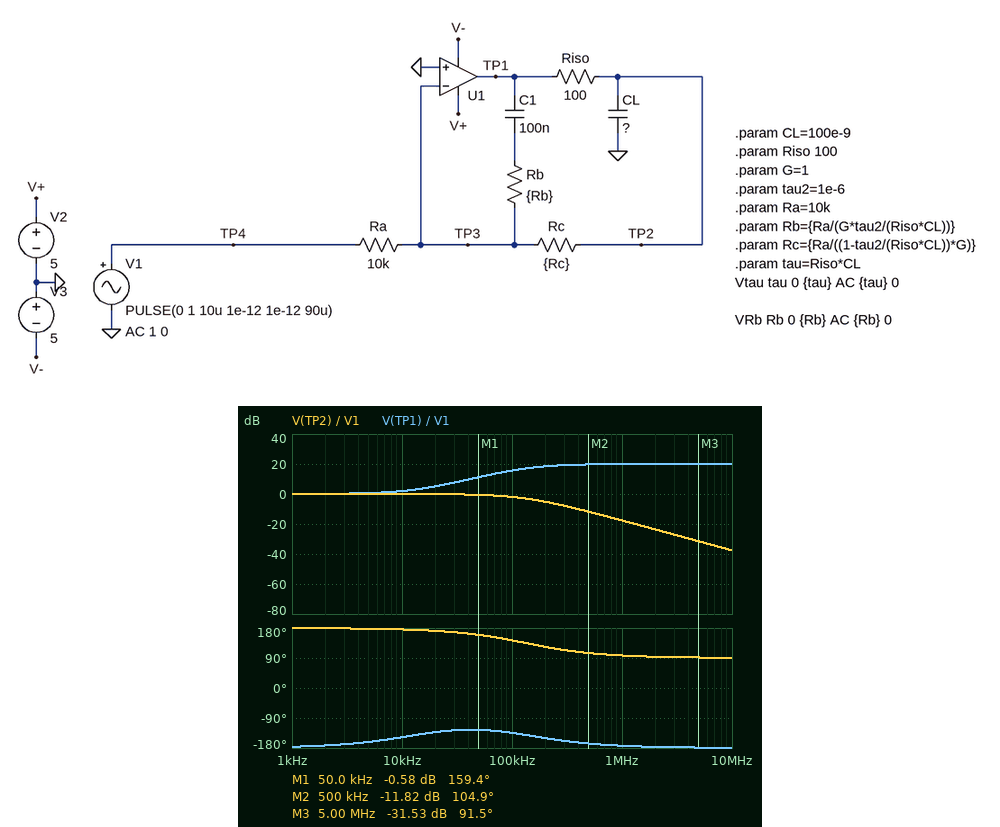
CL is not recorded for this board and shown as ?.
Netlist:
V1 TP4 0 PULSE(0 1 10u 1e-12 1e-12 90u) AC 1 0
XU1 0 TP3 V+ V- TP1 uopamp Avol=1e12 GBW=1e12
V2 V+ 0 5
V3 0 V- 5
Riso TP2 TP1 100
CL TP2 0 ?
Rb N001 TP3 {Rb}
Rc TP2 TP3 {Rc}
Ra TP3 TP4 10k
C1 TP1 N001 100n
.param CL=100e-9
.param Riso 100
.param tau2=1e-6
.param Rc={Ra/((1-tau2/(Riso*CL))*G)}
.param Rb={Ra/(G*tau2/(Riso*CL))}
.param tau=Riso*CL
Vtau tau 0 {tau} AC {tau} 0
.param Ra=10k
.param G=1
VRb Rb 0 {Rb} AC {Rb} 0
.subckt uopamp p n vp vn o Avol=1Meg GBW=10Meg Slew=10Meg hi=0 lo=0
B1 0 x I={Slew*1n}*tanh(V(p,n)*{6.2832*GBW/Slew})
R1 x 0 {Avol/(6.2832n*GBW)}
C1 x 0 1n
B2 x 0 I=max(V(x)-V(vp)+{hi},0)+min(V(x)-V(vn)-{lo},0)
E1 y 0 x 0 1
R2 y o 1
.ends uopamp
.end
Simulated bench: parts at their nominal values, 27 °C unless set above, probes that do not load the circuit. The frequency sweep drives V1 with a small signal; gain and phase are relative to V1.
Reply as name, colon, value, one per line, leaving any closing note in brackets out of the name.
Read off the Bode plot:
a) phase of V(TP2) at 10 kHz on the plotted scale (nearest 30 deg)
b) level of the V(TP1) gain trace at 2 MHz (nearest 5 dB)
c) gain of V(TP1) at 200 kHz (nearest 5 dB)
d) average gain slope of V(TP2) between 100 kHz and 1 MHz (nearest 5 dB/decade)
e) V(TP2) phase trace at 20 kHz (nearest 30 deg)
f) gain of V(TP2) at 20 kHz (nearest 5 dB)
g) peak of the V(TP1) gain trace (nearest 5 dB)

phase of V(TP2) at 10 kHz on the plotted scale: 180 deg
level of the V(TP1) gain trace at 2 MHz: 20 dB
gain of V(TP1) at 200 kHz: 20 dB
average gain slope of V(TP2) between 100 kHz and 1 MHz: -15 dB/decade
V(TP2) phase trace at 20 kHz: 180 deg
gain of V(TP2) at 20 kHz: 0 dB
peak of the V(TP1) gain trace: 20 dB
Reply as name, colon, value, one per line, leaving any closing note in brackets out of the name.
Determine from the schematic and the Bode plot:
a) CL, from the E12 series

CL, from the E12 series: 120 nF
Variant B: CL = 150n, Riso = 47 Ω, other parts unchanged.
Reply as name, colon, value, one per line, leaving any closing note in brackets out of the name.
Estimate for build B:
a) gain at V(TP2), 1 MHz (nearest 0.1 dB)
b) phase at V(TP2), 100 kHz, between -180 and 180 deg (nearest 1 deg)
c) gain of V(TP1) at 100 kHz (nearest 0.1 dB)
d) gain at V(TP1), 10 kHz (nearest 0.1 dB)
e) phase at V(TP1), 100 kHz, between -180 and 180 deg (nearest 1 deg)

gain at V(TP2), 1 MHz: -13.1 dB
phase at V(TP2), 100 kHz, between -180 and 180 deg: 156 deg
gain of V(TP1) at 100 kHz: 12.4 dB
gain at V(TP1), 10 kHz: 0.8 dB
phase at V(TP1), 100 kHz, between -180 and 180 deg: -127 deg
